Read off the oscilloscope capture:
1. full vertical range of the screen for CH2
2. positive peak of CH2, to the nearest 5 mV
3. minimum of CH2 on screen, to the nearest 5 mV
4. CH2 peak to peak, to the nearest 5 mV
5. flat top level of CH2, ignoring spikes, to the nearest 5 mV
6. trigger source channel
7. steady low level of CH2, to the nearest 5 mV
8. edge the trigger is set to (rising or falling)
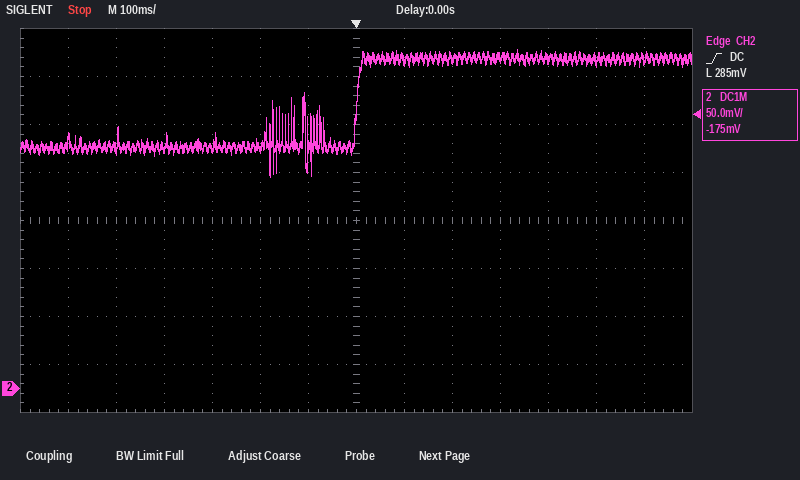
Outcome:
400 mV
355 mV
220 mV
135 mV
345 mV
CH2
250 mV
rising
